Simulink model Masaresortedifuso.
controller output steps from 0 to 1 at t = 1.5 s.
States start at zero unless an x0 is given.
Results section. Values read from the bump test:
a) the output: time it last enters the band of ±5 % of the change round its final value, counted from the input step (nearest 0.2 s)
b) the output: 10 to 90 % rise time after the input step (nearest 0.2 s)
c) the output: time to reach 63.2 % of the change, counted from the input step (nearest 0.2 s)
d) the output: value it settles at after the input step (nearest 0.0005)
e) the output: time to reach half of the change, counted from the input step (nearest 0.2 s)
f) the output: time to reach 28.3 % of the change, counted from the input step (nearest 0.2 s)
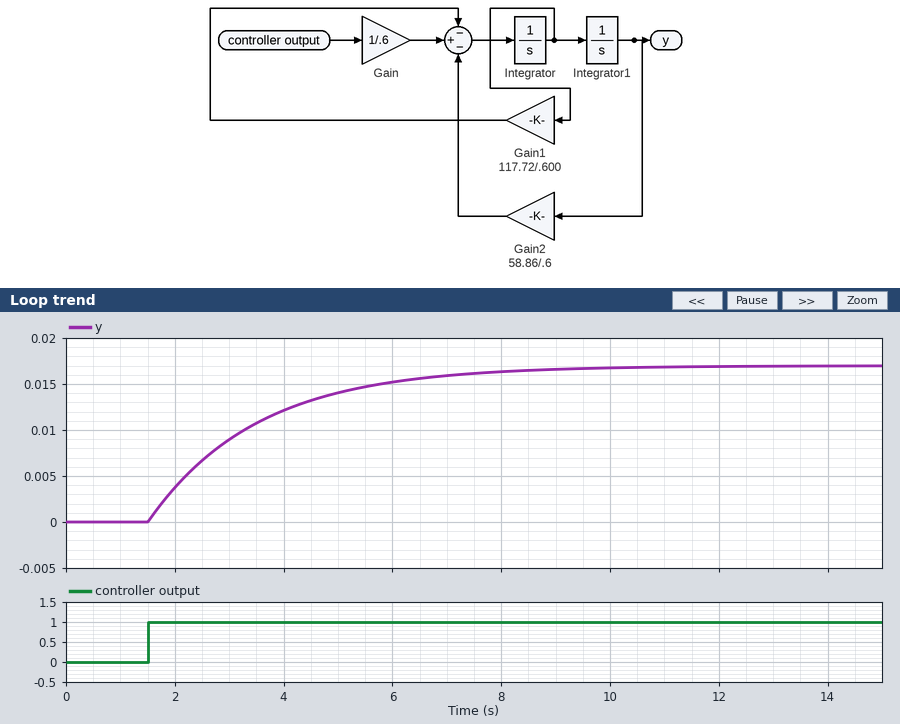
6.0 s
4.4 s
2.0 s
0.0170
1.4 s
0.6 s
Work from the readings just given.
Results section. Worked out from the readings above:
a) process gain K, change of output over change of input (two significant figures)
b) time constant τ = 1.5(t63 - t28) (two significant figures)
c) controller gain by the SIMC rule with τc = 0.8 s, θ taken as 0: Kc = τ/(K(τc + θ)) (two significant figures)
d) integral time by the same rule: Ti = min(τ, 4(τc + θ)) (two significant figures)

0.017
2.1 s
150
2.1 s
